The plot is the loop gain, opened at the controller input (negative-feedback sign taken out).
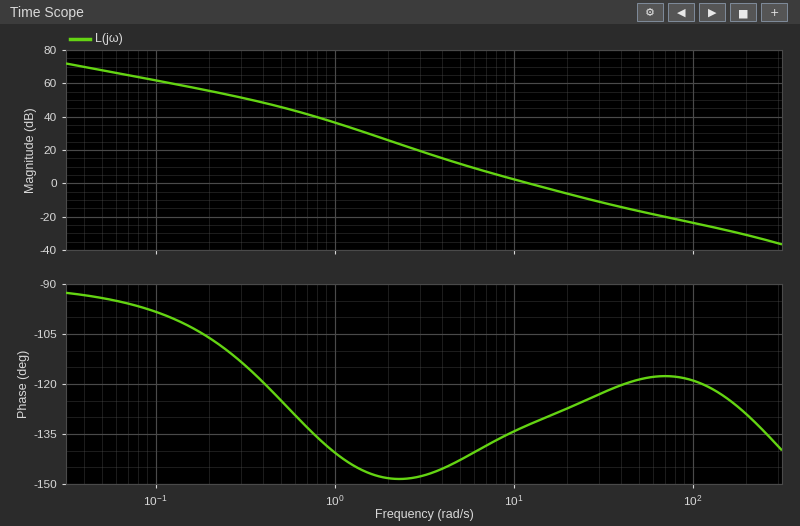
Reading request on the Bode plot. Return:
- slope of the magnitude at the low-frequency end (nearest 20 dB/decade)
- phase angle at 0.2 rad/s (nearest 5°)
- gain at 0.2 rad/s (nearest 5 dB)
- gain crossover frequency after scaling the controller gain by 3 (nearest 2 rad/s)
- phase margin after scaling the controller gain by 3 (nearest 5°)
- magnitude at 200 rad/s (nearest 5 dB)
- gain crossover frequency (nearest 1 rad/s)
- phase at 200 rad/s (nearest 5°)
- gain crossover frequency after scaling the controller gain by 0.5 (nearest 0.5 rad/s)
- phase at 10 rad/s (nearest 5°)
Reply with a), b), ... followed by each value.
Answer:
a) -20 dB/decade
b) -105°
c) 55 dB
d) 26 rad/s
e) 55°
f) -30 dB
g) 12 rad/s
h) -130°
i) 7.5 rad/s
j) -135°
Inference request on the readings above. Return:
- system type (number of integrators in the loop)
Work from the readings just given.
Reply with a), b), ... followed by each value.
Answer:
a) 1
